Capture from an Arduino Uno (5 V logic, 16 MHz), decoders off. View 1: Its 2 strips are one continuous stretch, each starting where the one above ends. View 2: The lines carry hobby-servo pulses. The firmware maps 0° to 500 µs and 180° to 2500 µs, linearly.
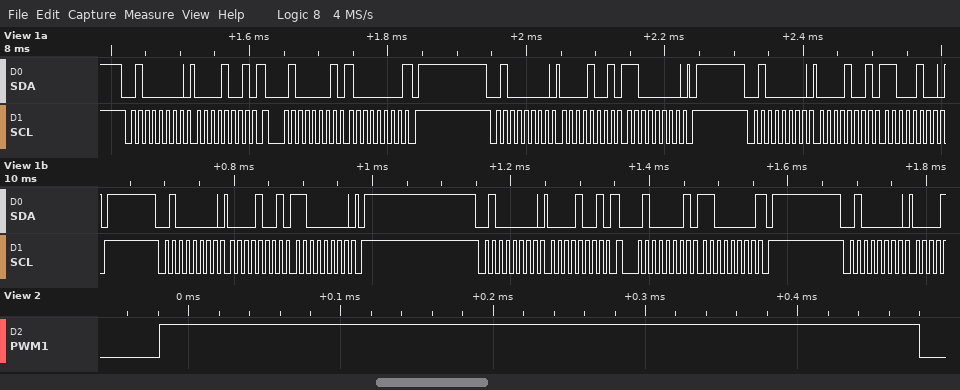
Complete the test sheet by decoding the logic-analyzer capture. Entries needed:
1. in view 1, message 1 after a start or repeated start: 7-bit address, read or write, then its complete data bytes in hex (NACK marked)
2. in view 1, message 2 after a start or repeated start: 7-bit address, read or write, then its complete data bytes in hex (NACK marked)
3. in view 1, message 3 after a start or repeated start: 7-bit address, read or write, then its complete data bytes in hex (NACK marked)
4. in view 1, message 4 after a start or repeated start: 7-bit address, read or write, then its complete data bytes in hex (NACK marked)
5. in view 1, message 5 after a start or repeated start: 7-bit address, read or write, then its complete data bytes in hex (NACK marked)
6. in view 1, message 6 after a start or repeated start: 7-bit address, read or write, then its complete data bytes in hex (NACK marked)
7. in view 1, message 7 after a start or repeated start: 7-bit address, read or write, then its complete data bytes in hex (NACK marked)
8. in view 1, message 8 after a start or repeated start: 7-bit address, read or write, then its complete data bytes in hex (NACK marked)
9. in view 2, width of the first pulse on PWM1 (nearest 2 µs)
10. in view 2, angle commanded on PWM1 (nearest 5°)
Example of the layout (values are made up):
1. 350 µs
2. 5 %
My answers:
1. 0x20 write: 09
2. 0x20 read: 80 NACK
3. 0x20 write: 09 C0
4. 0x20 write: 09 C4
5. 0x20 write: 09 C0
6. 0x20 write: 09
7. 0x20 read: C0 NACK
8. 0x20 write
9. 500 µs
10. 0°
